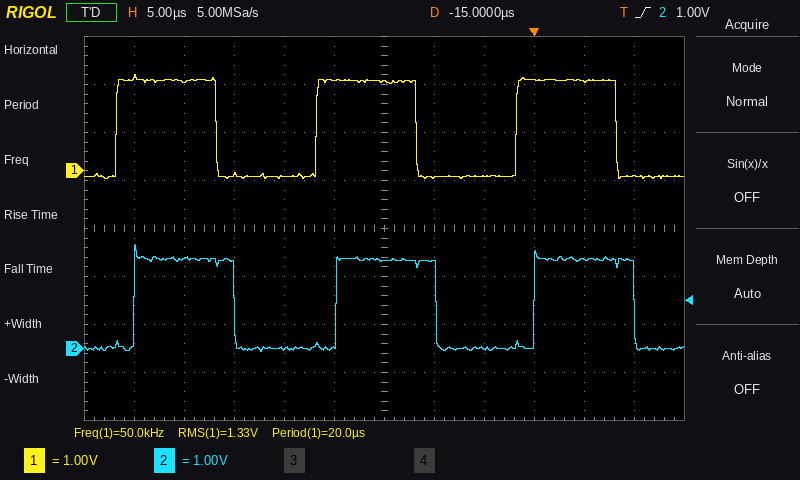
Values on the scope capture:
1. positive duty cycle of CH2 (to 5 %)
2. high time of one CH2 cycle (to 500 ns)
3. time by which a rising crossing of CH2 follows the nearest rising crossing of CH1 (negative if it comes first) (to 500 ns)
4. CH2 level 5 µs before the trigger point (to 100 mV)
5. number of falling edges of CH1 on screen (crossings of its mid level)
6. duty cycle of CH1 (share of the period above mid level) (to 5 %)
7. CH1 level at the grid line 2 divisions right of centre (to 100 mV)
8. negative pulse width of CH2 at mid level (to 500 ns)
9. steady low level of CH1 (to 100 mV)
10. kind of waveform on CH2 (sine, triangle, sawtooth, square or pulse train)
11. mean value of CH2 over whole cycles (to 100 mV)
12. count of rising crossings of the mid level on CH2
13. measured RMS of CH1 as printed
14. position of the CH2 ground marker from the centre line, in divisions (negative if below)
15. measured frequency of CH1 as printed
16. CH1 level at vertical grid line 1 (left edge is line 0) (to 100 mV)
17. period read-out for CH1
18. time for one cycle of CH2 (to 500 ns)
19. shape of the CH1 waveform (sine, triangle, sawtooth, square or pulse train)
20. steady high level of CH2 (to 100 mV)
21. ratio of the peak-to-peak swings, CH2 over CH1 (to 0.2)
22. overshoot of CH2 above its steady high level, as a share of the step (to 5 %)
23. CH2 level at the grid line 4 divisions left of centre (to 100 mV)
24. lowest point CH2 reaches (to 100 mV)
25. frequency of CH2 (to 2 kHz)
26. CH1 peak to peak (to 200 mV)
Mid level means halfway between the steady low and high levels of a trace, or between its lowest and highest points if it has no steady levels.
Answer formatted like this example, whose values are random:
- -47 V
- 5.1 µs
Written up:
- 50 %
- 10.0 µs
- +2.0 µs
- 0.0 V
- 3
- 50 %
- -100 mV
- 10.0 µs
- -100 mV
- square
- 900 mV
- 3
- 1.33 V
- -2.5 div
- 50.0 kHz
- 1.9 V
- 20.0 µs
- 20.0 µs
- square
- 1.9 V
- 1.0
- 15 %
- 1.9 V
- -100 mV
- 50 kHz
- 2.2 V
